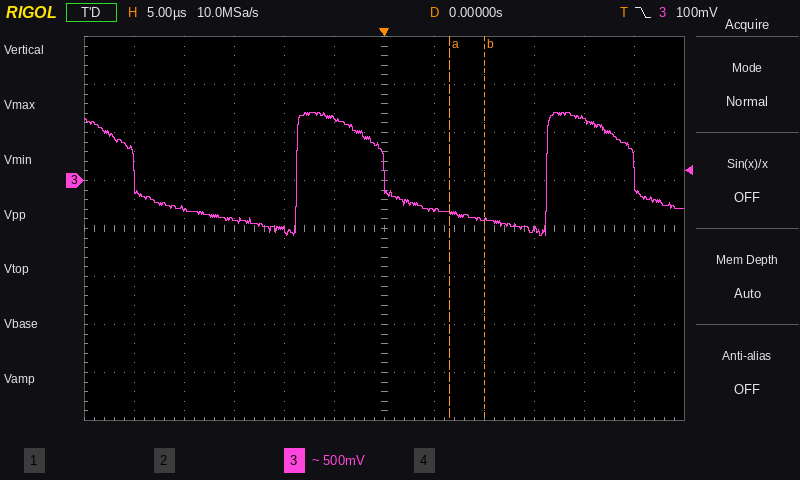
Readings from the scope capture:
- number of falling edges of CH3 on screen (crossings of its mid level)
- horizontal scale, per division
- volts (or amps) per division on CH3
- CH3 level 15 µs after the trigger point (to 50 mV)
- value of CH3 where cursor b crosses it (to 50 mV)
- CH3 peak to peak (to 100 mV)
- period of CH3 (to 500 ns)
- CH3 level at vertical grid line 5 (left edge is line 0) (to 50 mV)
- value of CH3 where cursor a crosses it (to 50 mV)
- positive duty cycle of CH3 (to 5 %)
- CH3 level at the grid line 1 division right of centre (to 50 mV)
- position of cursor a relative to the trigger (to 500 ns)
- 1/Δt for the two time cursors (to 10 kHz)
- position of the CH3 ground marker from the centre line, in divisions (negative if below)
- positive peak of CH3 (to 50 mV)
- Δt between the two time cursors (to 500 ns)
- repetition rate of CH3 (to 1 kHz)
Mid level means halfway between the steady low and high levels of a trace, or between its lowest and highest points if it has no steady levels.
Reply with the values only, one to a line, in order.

3
5 µs
500 mV
-500 mV
-400 mV
1.30 V
25.0 µs
650 mV
-350 mV
35 %
-300 mV
+6.5 µs
290 kHz
+1.0 div
700 mV
3.5 µs
40 kHz
